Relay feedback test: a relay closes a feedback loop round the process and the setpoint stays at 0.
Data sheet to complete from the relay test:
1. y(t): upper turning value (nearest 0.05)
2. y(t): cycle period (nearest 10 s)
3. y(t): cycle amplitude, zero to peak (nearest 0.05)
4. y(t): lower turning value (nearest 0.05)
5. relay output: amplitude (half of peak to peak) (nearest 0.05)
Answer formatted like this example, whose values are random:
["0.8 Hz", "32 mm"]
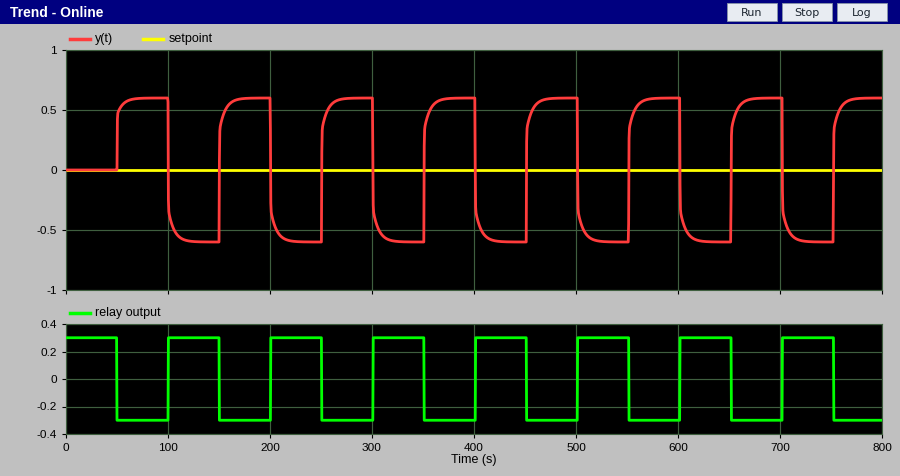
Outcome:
["0.60", "100 s", "0.60", "-0.60", "0.30"]
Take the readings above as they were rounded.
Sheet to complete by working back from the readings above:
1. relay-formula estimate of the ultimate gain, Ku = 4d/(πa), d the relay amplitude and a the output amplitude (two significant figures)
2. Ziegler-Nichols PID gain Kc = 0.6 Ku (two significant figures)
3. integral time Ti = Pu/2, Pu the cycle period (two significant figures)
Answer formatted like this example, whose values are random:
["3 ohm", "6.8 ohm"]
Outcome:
["0.64", "0.38", "50 s"]
